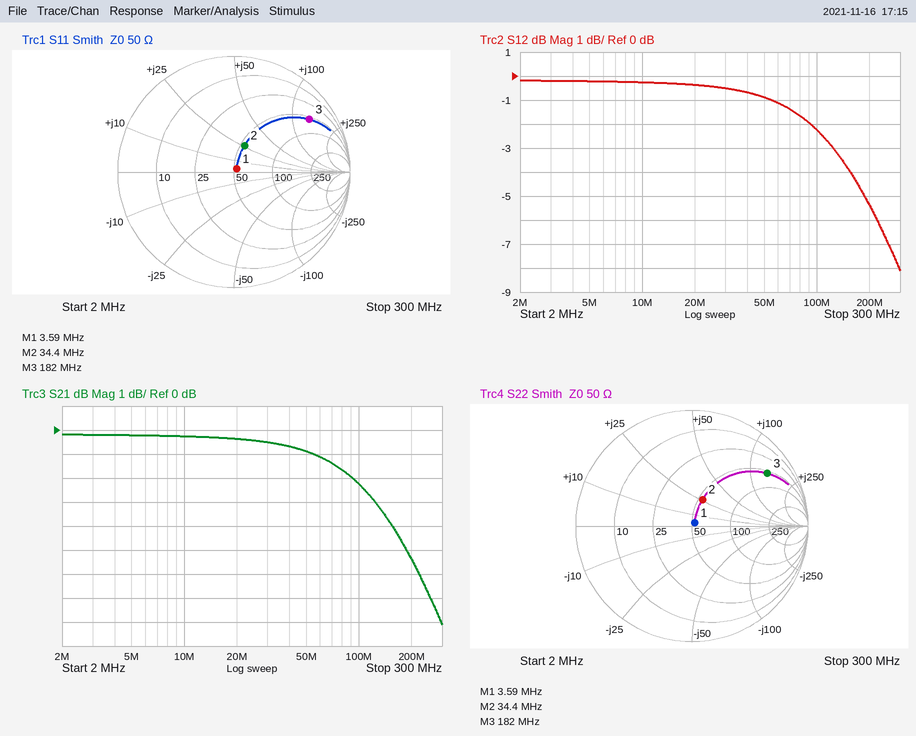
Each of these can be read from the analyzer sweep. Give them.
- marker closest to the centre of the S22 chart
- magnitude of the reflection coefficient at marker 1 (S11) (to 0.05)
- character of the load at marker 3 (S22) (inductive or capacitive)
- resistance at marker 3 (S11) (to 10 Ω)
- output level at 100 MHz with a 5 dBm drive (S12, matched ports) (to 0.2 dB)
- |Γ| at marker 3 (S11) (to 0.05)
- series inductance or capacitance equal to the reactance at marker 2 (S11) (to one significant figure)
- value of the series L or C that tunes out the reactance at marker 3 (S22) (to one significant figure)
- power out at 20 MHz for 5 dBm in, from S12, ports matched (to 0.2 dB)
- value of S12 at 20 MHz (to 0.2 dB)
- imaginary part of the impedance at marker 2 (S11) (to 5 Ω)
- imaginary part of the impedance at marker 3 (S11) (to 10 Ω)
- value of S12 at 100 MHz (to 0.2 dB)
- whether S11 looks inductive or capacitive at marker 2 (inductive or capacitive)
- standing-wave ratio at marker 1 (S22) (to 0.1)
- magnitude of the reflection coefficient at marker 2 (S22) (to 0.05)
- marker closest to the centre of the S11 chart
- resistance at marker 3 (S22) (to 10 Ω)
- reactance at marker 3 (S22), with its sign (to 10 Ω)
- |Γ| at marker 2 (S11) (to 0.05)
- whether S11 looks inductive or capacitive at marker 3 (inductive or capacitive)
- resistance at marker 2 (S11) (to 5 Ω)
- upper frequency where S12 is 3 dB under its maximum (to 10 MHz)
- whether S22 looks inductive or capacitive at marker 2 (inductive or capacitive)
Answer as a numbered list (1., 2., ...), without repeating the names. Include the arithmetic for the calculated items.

1. marker 1
2. 0.05
3. inductive
4. 60 Ω
5. 5 dBm + (-2.2 dB) = 2.8 dBm
6. 0.80
7. L = 25 Ω/(2π × 34.4 MHz) ≈ 116 nH, so 100 nH to one significant figure
8. C = 1/(2π × 182 MHz × 140 Ω) ≈ 6 pF
9. 5 dBm + (-0.4 dB) = 4.6 dBm
10. -0.4 dB
11. +25 Ω
12. +140 Ω
13. -2.2 dB
14. inductive
15. 1.1
16. 0.25
17. marker 1
18. 60 Ω
19. +140 Ω
20. 0.25
21. inductive
22. 55 Ω
23. 130 MHz
24. inductive
